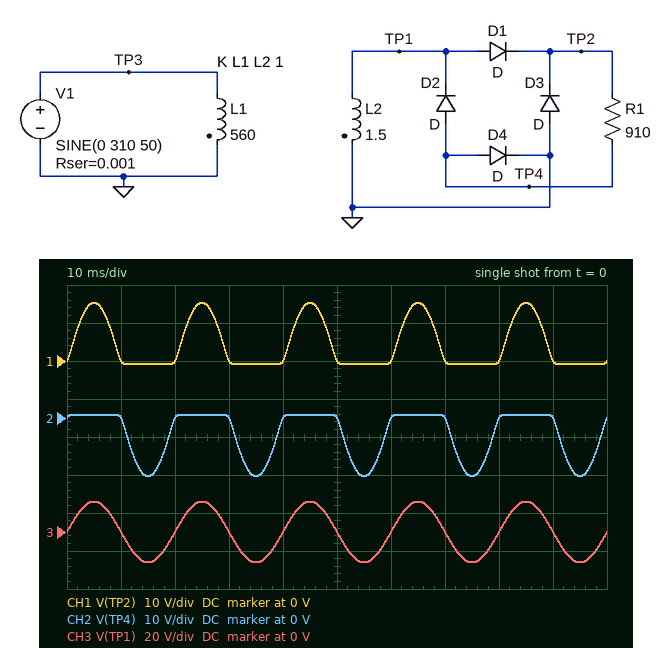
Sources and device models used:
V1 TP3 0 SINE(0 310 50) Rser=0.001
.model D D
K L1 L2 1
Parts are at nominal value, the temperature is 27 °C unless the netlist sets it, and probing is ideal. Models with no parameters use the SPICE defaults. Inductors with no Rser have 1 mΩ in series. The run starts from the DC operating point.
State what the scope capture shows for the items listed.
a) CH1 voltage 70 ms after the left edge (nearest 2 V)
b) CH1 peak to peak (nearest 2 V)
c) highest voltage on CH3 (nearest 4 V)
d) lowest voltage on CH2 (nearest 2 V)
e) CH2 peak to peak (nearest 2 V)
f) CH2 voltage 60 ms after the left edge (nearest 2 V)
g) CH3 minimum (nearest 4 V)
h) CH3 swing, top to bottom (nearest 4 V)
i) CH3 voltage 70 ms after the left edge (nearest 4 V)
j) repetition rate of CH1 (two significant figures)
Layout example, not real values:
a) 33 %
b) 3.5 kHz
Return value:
a) 0 V
b) 16 V
c) 16 V
d) -16 V
e) 16 V
f) 0 V
g) -16 V
h) 32 V
i) 0 V
j) 50 Hz
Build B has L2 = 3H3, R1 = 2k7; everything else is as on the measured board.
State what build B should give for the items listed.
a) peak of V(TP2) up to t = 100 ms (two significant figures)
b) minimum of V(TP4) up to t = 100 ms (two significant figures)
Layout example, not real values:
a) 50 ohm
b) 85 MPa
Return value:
a) 23 V
b) -23 V
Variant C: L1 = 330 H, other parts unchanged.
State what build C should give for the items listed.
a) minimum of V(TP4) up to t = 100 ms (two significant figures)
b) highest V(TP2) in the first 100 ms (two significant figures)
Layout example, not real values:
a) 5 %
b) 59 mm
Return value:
a) -20 V
b) 20 V
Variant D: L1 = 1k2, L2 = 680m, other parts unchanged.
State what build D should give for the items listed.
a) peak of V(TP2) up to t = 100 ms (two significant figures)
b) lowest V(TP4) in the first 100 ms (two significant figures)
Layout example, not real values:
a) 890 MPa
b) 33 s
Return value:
a) 6.7 V
b) -6.7 V
